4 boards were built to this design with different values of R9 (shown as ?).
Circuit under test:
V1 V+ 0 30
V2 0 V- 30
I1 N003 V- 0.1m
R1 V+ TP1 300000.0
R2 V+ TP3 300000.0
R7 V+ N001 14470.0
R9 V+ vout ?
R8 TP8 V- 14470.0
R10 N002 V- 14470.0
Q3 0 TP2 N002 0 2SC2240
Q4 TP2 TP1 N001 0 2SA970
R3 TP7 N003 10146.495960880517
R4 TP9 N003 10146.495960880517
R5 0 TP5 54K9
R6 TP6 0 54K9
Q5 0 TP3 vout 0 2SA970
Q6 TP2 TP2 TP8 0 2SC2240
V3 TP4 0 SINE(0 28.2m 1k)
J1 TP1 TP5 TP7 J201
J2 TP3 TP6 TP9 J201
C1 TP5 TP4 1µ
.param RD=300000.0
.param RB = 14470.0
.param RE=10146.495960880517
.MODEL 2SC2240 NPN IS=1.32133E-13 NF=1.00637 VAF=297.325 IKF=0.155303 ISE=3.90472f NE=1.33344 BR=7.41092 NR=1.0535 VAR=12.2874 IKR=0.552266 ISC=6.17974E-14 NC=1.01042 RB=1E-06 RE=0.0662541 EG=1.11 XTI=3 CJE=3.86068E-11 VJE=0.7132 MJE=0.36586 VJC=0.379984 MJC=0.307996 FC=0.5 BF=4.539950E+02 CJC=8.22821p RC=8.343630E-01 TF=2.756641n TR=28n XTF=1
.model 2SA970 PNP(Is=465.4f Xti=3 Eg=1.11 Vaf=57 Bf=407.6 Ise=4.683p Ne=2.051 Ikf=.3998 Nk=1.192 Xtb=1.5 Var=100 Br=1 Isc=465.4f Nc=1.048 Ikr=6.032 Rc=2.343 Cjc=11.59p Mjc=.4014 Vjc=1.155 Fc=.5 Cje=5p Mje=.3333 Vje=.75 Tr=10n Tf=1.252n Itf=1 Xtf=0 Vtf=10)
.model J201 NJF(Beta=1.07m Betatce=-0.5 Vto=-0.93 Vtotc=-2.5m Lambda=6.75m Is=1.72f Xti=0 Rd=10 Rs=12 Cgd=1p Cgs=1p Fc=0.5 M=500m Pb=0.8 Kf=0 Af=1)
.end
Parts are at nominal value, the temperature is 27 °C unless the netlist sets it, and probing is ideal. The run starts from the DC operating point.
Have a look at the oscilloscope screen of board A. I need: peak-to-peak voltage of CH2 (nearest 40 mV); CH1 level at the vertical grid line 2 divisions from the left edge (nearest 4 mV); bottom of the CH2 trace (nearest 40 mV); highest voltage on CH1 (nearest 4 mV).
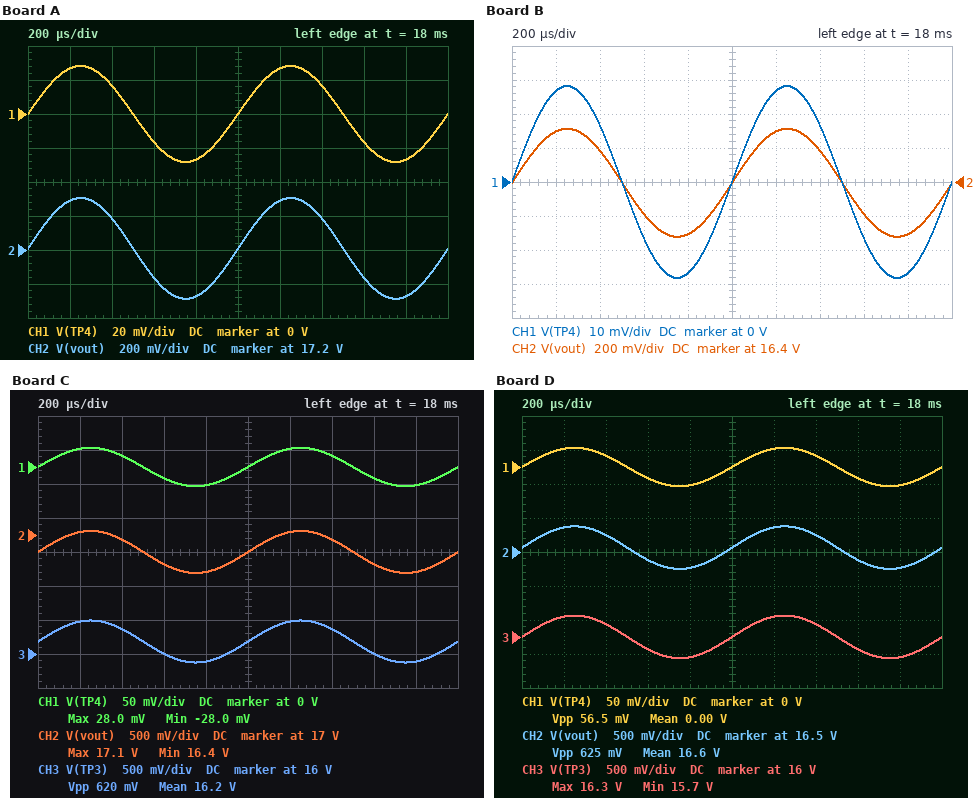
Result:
600 mV
16 mV
16.92 V
28 mV
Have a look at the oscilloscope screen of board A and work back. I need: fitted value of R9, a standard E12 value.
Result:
4.7 kΩ
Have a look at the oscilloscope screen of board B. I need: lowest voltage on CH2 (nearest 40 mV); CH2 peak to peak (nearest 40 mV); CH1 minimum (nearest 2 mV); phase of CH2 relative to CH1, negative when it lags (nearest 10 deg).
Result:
16.08 V
640 mV
-28 mV
0 deg
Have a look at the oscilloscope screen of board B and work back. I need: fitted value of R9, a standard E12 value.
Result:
10 kΩ
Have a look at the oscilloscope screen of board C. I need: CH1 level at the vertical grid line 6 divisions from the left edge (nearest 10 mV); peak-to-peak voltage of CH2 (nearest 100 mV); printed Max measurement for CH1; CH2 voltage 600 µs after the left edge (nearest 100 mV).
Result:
30 mV
600 mV
28.0 mV
16.6 V
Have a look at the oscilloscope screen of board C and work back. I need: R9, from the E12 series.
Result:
6.8 kΩ
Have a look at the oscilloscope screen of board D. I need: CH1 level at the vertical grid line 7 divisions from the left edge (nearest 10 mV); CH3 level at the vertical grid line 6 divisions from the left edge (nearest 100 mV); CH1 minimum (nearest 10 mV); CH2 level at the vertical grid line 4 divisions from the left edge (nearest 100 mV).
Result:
20 mV
16.3 V
-30 mV
16.3 V
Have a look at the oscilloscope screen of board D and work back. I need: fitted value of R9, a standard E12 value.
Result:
8.2 kΩ
